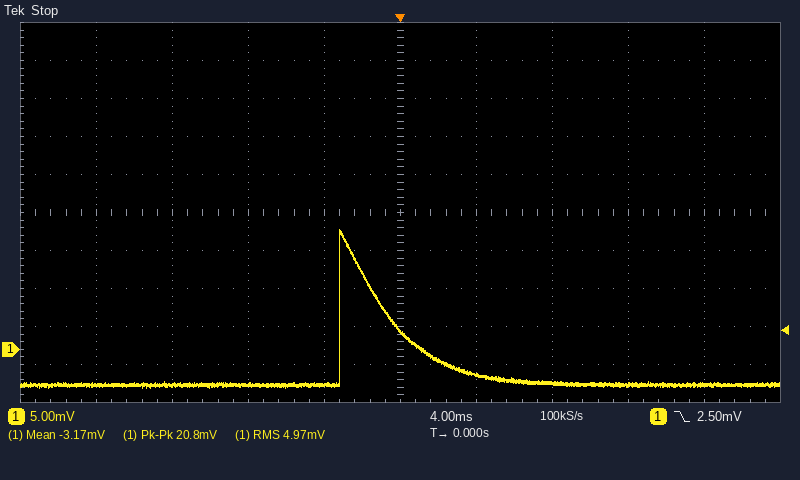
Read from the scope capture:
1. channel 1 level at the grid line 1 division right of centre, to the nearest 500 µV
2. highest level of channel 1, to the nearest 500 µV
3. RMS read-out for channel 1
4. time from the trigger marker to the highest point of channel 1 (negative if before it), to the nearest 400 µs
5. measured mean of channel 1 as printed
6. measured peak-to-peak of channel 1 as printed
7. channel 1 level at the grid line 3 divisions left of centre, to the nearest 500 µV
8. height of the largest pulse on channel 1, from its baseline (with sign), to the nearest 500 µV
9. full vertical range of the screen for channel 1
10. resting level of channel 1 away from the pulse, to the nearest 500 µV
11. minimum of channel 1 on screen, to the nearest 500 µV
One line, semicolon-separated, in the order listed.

-3.5 mV; 16.0 mV; 4.97 mV; -3.2 ms; -3.17 mV; 20.8 mV; -4.5 mV; +20.5 mV; 50 mV; -4.5 mV; -5.0 mV
